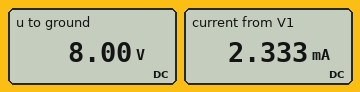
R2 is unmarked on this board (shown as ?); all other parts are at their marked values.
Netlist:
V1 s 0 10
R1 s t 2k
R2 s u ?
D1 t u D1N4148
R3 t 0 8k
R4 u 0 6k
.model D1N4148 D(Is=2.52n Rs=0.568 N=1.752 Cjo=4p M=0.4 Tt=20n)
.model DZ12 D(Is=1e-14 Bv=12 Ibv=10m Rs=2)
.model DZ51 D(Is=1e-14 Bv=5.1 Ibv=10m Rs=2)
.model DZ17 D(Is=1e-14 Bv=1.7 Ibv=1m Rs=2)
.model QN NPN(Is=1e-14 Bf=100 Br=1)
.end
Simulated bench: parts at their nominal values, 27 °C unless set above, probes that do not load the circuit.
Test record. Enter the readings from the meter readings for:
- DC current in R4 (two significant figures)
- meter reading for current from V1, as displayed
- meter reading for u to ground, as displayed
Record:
1.3 mA
2.333 mA
8.00 V
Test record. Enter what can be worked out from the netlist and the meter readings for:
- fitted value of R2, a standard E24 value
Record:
1.5 kΩ
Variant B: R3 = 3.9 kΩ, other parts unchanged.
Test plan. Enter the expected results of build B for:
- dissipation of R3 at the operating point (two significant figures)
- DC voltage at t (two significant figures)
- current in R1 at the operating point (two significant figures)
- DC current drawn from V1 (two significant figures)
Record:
11 mW
6.6 V
1.7 mA
3.0 mA
